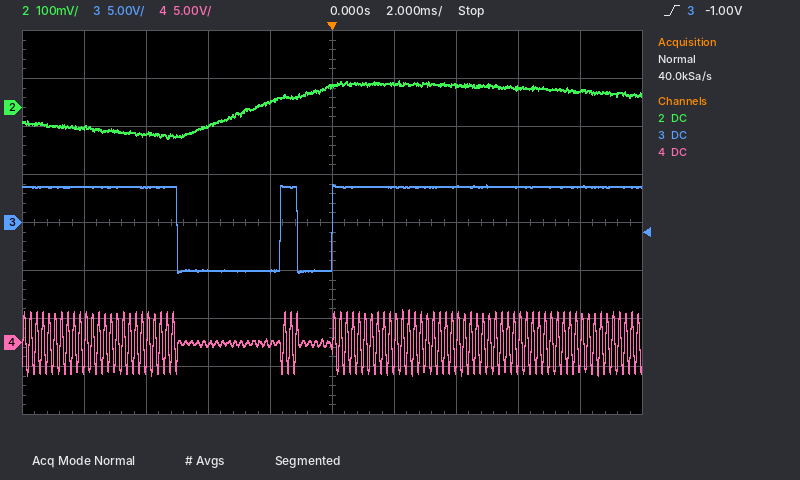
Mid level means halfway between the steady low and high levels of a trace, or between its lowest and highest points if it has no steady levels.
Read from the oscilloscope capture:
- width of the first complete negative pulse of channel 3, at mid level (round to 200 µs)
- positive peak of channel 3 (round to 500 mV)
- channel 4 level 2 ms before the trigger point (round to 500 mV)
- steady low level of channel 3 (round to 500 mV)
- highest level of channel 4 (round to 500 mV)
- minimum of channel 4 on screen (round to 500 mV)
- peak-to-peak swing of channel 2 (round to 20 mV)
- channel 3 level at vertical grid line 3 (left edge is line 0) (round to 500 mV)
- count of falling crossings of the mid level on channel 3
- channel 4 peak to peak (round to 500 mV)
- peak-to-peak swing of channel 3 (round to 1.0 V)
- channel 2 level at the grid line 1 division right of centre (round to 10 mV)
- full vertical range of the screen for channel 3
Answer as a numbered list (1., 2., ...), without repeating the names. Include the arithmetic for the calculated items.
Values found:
1. 3.4 ms
2. 4.0 V
3. 0.0 V
4. -5.0 V
5. 3.5 V
6. -3.5 V
7. 120 mV
8. -5.0 V
9. 2
10. 3.5 V − (-3.5 V) = 7.0 V
11. 9.0 V
12. 50 mV
13. 40 V
